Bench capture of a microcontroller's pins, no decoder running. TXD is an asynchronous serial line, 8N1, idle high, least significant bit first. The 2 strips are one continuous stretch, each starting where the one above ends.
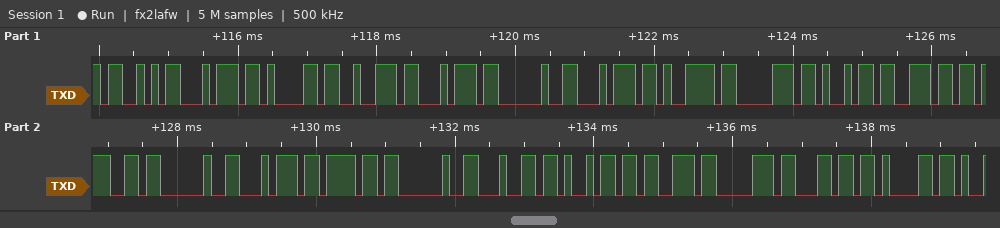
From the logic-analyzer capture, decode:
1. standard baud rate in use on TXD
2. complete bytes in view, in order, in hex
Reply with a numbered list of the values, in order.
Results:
1. 9600 baud
2. 53 74 61 72 74 20 74 79 70 69 6E 67 20 74 6F 20 64 69 73 70 6C 61
